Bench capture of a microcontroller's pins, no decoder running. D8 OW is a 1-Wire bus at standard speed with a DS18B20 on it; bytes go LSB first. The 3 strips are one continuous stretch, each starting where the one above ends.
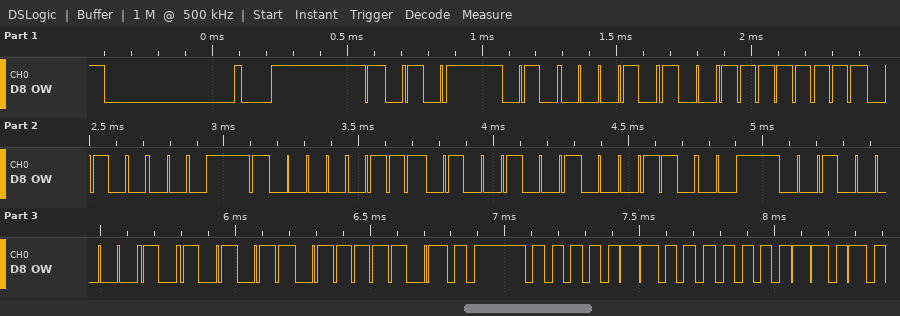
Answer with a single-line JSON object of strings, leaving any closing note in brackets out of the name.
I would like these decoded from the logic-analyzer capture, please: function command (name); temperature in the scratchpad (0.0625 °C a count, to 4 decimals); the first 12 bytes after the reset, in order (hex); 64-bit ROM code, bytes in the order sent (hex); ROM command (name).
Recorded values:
{"function command": "Read Scratchpad", "temperature in the scratchpad": "24.0000 °C", "the first 12 bytes after the reset, in order": "55 28 FF 82 E0 92 18 04 D5 BE 80 01", "64-bit ROM code, bytes in the order sent": "28 FF 82 E0 92 18 04 D5", "ROM command": "Match ROM"}
